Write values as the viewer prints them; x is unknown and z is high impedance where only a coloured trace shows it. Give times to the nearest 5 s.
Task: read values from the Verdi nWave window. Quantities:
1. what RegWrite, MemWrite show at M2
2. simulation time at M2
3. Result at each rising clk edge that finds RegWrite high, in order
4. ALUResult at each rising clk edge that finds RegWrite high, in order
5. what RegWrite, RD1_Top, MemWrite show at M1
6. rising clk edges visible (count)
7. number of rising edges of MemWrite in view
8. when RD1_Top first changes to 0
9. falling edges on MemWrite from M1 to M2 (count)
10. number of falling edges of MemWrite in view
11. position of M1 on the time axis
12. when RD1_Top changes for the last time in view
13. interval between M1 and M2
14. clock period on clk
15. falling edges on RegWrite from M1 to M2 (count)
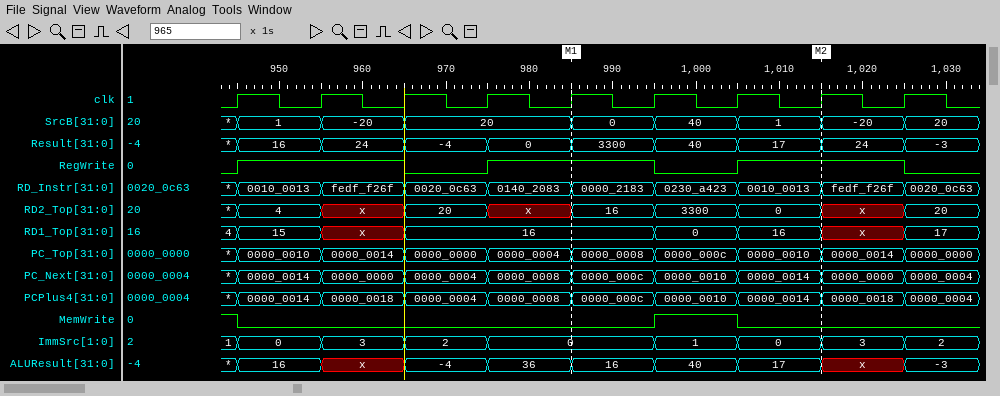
RegWrite=1, MemWrite=0
1015 s
16, 24, 0, 3300, 17, 24
16, x, 36, 16, 17, x
RegWrite=1, RD1_Top=16, MemWrite=0
9
1
995 s
1
2
985 s
1025 s
30 s
10 s
1
